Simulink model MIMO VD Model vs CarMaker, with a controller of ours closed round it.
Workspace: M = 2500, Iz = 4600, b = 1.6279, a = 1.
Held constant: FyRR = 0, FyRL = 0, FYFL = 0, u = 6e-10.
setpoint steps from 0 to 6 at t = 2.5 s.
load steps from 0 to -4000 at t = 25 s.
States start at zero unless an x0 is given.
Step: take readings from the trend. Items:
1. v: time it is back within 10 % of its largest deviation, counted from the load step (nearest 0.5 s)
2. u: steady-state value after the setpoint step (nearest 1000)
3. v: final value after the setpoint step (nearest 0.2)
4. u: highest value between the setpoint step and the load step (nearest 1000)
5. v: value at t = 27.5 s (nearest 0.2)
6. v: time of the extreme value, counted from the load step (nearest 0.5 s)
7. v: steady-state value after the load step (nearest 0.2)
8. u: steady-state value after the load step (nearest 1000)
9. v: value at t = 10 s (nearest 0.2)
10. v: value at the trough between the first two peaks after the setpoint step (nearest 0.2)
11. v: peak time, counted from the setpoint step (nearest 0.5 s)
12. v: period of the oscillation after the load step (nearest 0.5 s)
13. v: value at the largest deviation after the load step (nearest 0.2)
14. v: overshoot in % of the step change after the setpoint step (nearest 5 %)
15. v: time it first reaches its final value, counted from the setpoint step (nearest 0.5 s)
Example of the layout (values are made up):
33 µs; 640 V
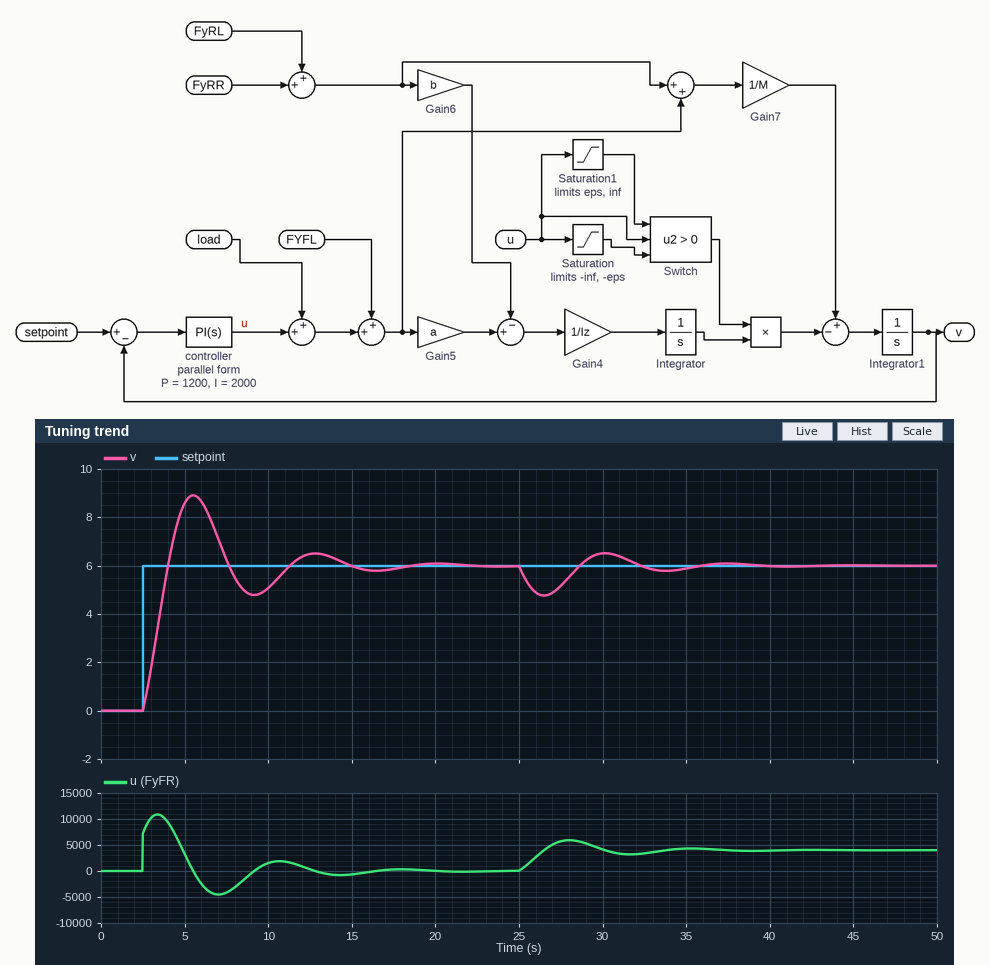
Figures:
10.0 s; 0; 6.0; 11000; 5.2; 1.5 s; 6.0; 4000; 5.0; 4.8; 3.0 s; 7.5 s; 4.8; 50 %; 1.5 s
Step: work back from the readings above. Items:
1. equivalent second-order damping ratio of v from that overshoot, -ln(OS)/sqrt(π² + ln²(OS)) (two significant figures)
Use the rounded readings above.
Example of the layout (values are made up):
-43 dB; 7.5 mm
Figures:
0.22
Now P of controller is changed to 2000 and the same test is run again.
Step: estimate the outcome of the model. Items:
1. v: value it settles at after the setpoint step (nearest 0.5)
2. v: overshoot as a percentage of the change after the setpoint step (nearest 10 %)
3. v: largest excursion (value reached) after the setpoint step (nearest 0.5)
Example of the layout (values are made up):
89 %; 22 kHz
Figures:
6.0; 30 %; 8.0
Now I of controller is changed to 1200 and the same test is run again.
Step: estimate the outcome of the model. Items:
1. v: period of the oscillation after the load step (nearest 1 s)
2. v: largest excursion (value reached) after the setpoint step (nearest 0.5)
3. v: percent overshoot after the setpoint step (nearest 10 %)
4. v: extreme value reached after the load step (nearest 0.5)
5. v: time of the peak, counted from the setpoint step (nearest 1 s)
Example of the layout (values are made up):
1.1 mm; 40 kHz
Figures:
10 s; 8.5; 40 %; 4.5; 4 s
